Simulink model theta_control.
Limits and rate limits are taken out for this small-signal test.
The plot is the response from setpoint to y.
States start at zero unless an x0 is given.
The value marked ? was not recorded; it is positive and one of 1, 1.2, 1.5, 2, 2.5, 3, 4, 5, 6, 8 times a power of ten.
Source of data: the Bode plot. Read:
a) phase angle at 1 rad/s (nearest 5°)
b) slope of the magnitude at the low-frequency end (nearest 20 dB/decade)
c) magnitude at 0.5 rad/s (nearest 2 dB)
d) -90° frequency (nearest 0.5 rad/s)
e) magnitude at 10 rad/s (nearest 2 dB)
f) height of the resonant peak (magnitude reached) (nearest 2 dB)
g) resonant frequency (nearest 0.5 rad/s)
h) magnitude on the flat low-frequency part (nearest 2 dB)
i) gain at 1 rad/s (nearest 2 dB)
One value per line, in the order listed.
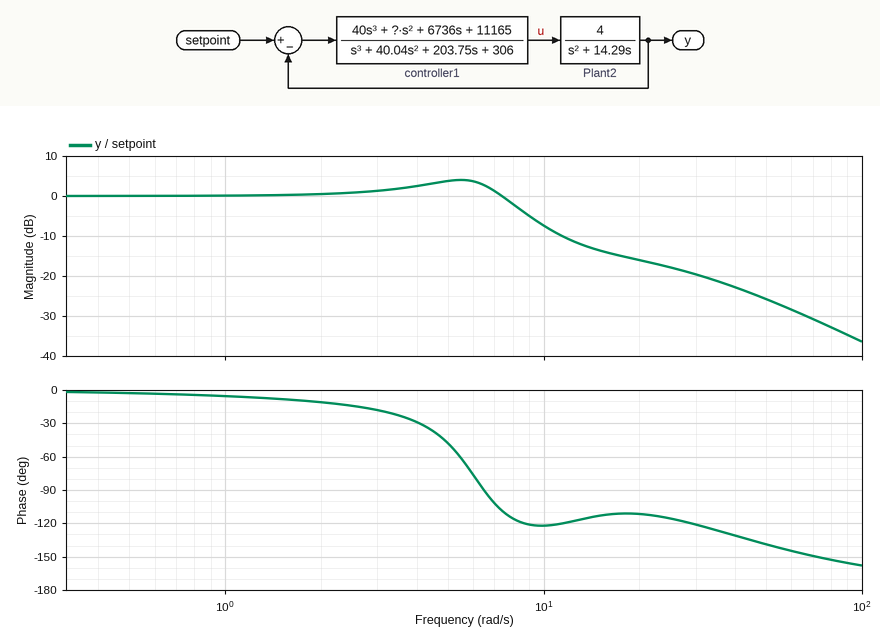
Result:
-5°
0 dB/decade
0 dB
6.5 rad/s
-8 dB
4 dB
5.5 rad/s
0 dB
0 dB
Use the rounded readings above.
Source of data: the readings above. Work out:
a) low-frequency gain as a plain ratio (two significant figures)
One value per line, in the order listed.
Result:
1.0
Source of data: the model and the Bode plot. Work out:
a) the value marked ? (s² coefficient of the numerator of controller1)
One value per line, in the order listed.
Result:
600
